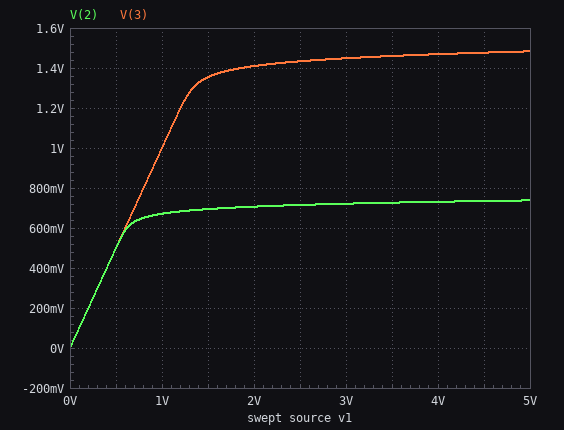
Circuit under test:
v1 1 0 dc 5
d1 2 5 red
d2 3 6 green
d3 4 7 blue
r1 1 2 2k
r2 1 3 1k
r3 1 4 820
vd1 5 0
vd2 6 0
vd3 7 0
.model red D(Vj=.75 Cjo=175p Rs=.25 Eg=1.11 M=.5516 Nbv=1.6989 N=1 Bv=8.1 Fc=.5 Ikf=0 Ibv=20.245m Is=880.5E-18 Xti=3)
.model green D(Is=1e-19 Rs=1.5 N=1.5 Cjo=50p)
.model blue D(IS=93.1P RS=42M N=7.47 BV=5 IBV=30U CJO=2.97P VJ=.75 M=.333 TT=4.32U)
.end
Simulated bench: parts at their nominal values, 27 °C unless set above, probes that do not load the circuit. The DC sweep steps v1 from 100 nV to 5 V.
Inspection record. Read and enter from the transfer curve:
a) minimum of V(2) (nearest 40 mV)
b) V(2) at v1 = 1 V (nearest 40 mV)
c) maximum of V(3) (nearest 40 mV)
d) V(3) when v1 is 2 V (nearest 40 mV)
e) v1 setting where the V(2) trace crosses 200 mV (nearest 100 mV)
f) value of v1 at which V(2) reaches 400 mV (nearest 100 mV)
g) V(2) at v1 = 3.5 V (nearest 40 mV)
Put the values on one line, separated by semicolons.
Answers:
0 V; 680 mV; 1.48 V; 1.40 V; 200 mV; 400 mV; 720 mV
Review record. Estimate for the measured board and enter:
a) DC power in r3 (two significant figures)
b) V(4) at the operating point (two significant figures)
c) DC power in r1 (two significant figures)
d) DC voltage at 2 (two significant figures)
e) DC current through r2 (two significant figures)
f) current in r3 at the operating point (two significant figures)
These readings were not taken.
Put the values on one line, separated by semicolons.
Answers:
3.6 mW; 3.3 V; 9.1 mW; 740 mV; 3.5 mA; 2.1 mA
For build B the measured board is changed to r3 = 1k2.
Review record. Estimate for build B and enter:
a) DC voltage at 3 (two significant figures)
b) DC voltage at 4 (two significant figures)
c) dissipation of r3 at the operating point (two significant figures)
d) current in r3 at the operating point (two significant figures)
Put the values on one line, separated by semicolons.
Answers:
1.5 V; 3.2 V; 2.7 mW; 1.5 mA
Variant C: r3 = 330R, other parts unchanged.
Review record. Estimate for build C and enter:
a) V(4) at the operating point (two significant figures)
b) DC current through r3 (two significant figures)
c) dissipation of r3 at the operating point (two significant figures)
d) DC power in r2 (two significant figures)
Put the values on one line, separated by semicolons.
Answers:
3.4 V; 4.8 mA; 7.5 mW; 12 mW
